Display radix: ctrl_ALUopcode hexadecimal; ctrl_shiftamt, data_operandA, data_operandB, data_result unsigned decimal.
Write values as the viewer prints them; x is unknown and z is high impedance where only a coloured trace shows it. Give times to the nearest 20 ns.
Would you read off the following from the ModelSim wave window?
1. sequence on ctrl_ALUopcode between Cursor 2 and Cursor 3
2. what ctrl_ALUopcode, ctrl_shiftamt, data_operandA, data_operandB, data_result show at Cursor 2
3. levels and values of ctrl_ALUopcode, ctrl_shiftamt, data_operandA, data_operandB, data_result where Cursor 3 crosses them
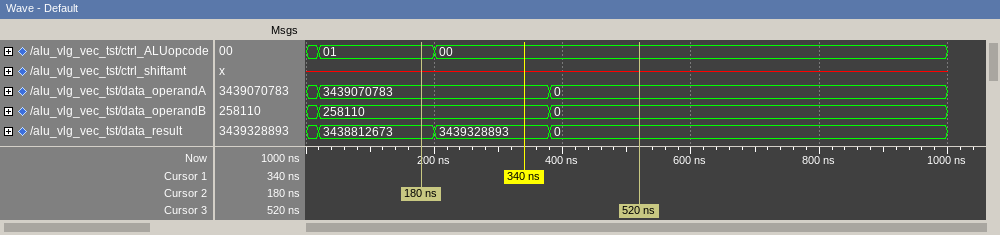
01, 00
ctrl_ALUopcode=01, ctrl_shiftamt=x, data_operandA=3439070783, data_operandB=258110, data_result=3438812673
ctrl_ALUopcode=00, ctrl_shiftamt=x, data_operandA=0, data_operandB=0, data_result=0
